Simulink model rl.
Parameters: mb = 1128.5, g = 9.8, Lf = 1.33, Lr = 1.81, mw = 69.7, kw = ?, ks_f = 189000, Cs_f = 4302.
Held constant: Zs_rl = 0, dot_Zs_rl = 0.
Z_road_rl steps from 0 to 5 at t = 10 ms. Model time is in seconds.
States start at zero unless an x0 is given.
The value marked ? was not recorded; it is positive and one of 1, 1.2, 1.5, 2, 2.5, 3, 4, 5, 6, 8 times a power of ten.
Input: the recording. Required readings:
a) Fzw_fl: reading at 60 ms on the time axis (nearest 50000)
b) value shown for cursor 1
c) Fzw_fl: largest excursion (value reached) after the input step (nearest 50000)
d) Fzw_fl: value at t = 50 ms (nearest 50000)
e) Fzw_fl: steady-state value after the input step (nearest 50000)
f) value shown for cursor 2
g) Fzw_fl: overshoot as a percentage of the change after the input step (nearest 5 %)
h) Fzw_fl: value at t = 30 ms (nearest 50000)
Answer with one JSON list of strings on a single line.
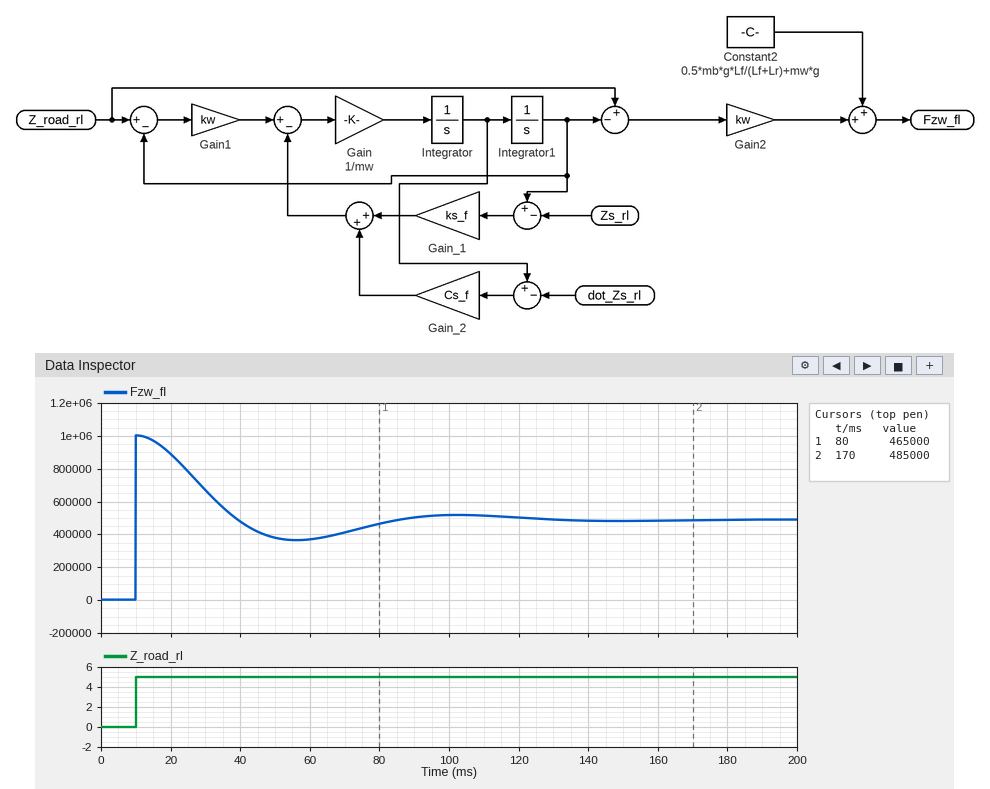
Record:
["350000", "465000", "1000000", "400000", "500000", "485000", "105 %", "650000"]
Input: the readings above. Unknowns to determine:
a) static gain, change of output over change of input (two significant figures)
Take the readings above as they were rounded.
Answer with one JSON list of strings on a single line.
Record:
["100000"]
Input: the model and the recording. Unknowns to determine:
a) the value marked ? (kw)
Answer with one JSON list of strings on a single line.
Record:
["200000"]
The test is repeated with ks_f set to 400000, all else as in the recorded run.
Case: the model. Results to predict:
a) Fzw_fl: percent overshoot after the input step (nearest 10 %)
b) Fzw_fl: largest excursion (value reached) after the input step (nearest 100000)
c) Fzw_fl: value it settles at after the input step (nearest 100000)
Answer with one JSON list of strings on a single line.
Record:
["50 %", "1000000", "700000"]
